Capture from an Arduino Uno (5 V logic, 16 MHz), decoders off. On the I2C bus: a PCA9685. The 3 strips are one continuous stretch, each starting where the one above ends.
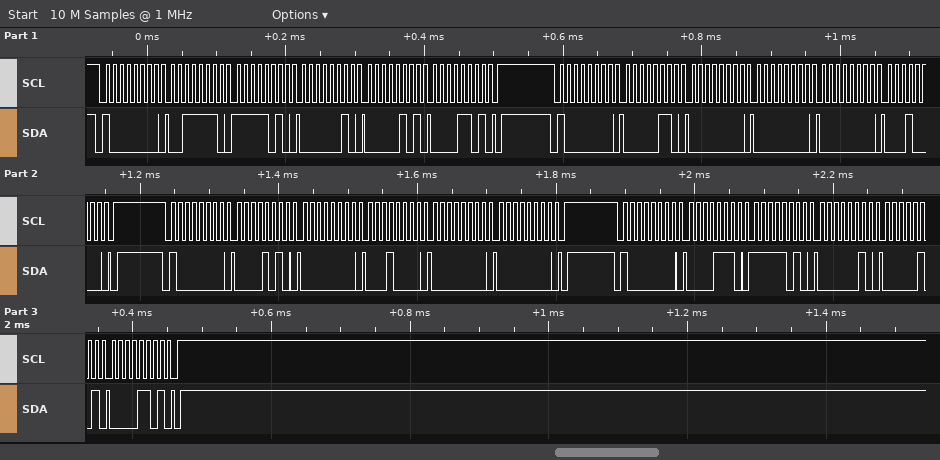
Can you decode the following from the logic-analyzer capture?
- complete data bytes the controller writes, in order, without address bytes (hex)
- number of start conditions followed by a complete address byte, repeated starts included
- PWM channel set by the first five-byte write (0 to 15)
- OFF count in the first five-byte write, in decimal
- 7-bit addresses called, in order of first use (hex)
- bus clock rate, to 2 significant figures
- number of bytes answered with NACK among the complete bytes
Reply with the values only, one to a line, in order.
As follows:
3E FA 02 05 0D 06 00 00 00 10 0A 00 10 00 00 0E FA 02 05 0D
4
14
3333
0x40
100 kHz
0
